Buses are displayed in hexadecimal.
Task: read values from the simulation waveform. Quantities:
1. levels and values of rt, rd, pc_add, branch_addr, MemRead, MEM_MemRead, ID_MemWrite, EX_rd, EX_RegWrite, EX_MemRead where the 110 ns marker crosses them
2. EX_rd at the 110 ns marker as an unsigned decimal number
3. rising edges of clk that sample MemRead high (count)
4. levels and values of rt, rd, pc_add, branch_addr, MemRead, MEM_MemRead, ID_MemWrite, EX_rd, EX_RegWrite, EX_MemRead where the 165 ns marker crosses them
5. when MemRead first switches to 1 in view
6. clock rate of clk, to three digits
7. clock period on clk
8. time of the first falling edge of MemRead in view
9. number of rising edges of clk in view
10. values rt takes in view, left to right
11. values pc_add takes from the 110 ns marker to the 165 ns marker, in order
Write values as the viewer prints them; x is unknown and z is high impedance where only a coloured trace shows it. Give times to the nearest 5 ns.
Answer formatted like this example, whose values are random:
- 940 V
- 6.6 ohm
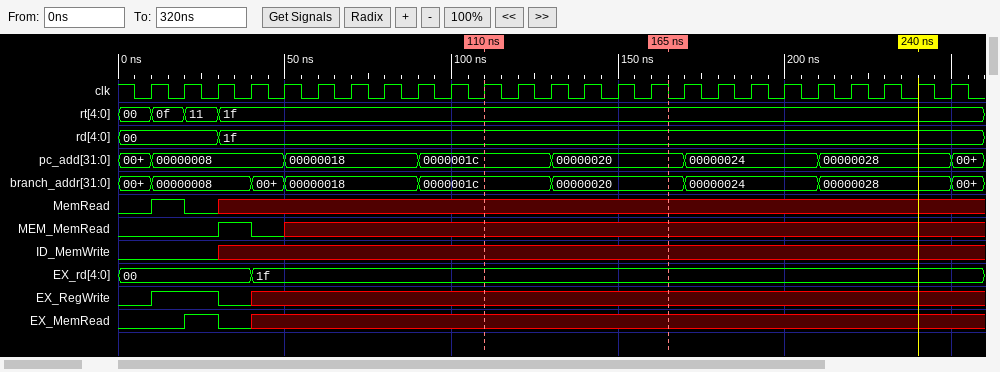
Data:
- rt=1f, rd=1f, pc_add=0000001c, branch_addr=0000001c, MemRead=x, MEM_MemRead=x, ID_MemWrite=x, EX_rd=1f, EX_RegWrite=x, EX_MemRead=x
- 31
- 1
- rt=1f, rd=1f, pc_add=00000020, branch_addr=00000020, MemRead=x, MEM_MemRead=x, ID_MemWrite=x, EX_rd=1f, EX_RegWrite=x, EX_MemRead=x
- 10 ns
- 100 MHz
- 10 ns
- 20 ns
- 25
- 00, 0f, 11, 1f
- 0000001c, 00000020
